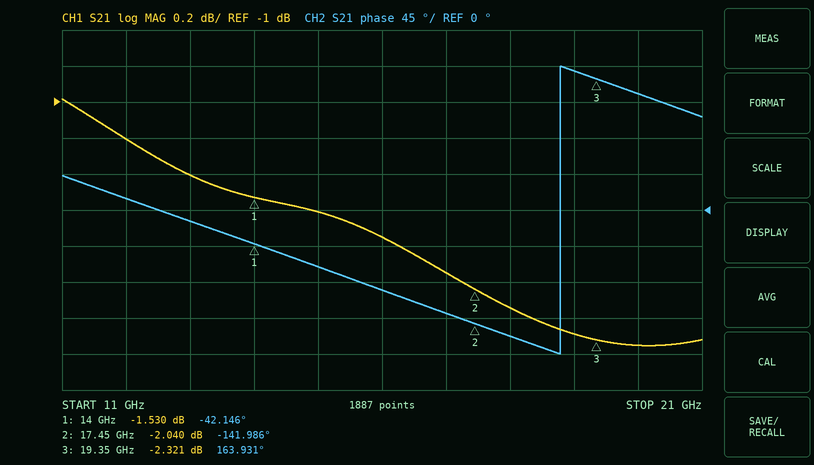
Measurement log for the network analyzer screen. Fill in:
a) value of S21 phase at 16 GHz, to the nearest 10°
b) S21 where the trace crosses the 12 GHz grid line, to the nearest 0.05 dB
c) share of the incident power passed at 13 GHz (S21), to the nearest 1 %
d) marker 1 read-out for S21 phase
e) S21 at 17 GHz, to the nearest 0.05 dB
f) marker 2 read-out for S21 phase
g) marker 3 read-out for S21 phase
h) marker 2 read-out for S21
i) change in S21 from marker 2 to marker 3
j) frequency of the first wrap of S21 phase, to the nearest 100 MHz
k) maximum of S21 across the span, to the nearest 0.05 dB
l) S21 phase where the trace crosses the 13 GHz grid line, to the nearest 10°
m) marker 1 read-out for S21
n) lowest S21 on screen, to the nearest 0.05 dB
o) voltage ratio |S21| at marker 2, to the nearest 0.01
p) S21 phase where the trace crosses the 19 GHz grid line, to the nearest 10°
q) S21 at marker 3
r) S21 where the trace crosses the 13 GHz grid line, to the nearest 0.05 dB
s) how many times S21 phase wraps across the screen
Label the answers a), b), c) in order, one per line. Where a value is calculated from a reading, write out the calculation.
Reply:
a) -100°
b) -1.20 dB
c) 10^(-1.4/10) ≈ 72 %
d) -42.146°
e) -1.95 dB
f) -141.986°
g) 163.931°
h) -2.040 dB
i) -2.321 − (-2.04) = -0.281 dB
j) 18.8 GHz
k) -1.00 dB
l) -10°
m) -1.530 dB
n) -2.35 dB
o) 10^(-2.04/20) ≈ 0.79
p) 170°
q) -2.321 dB
r) -1.40 dB
s) 1
